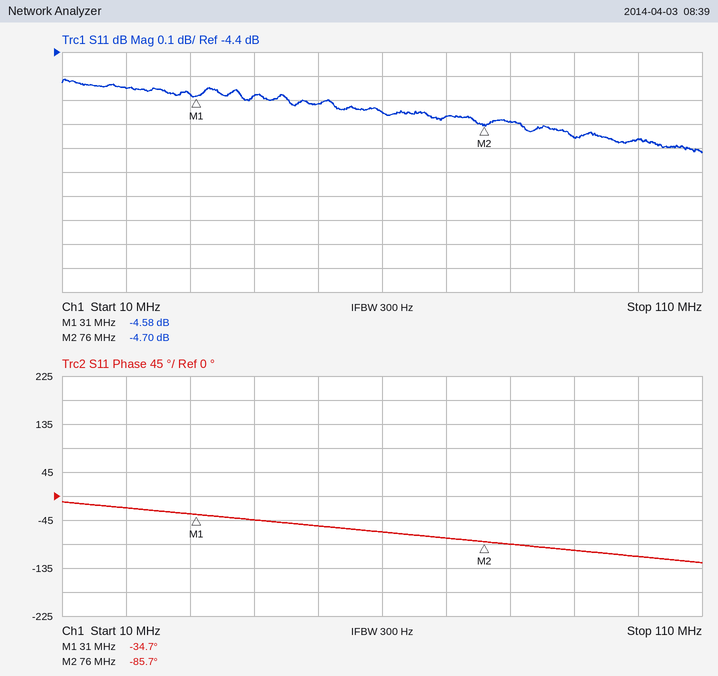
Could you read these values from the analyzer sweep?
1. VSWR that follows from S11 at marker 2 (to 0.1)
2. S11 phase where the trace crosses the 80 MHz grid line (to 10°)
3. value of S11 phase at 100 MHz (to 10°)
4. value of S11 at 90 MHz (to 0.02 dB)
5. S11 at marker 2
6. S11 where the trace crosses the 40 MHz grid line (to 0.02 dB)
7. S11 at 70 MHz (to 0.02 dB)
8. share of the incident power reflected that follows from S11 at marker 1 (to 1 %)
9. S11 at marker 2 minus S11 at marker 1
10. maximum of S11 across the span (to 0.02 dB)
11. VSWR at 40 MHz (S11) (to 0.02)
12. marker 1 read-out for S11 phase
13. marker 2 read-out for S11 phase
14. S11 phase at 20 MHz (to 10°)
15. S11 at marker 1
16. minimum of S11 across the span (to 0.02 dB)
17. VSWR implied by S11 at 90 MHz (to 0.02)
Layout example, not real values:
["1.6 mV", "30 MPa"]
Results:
["3.8", "-90°", "-110°", "-4.76 dB", "-4.70 dB", "-4.58 dB", "-4.66 dB", "35 %", "-0.12 dB", "-4.52 dB", "3.88", "-34.7°", "-85.7°", "-20°", "-4.58 dB", "-4.82 dB", "3.74"]
